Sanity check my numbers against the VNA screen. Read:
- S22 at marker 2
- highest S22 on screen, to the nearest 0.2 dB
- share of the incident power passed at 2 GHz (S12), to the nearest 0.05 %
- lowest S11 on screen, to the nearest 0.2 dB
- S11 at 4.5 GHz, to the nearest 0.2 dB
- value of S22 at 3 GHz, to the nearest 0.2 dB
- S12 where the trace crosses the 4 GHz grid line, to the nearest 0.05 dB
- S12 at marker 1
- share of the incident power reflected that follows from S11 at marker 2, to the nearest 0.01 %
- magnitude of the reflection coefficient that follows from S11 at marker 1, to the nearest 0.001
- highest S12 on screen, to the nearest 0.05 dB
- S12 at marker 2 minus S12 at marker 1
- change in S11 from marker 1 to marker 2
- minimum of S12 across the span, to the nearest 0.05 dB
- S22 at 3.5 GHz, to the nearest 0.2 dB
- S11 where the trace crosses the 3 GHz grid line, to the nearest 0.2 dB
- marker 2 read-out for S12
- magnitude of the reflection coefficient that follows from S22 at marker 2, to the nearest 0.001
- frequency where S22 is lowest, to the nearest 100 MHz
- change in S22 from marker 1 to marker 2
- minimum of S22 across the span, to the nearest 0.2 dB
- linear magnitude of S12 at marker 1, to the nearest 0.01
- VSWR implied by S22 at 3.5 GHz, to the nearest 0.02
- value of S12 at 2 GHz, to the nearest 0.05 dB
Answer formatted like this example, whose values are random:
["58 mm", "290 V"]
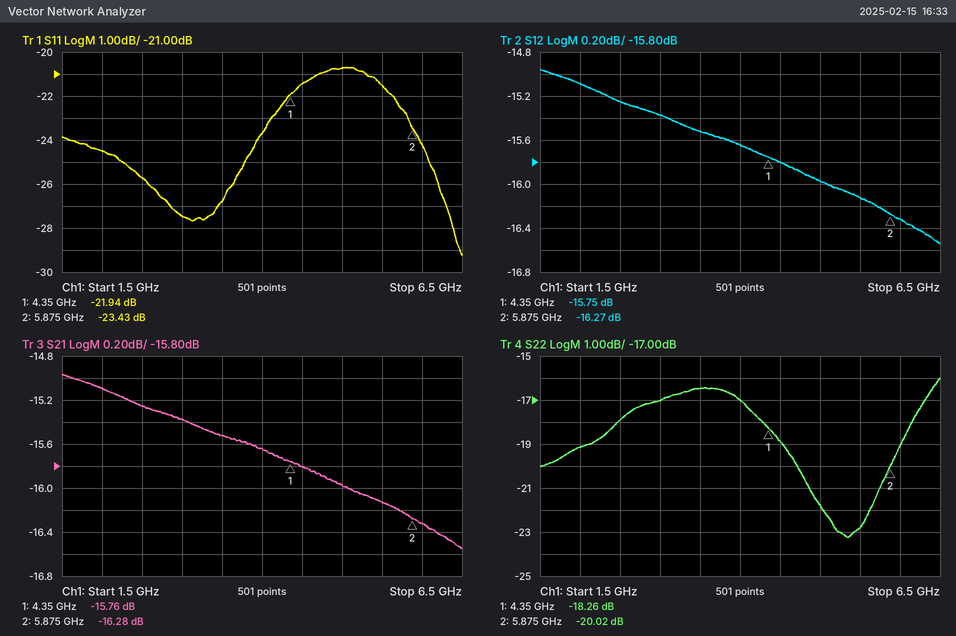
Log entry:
["-20.02 dB", "-16.0 dB", "3.10 %", "-29.2 dB", "-21.4 dB", "-17.0 dB", "-15.65 dB", "-15.75 dB", "0.45 %", "0.080", "-14.95 dB", "-0.52 dB", "-1.49 dB", "-16.55 dB", "-16.4 dB", "-27.4 dB", "-16.27 dB", "0.100", "5.3 GHz", "-1.76 dB", "-23.2 dB", "0.16", "1.36", "-15.10 dB"]
